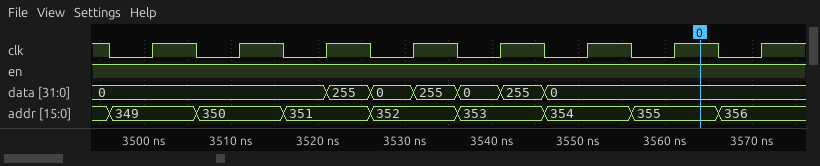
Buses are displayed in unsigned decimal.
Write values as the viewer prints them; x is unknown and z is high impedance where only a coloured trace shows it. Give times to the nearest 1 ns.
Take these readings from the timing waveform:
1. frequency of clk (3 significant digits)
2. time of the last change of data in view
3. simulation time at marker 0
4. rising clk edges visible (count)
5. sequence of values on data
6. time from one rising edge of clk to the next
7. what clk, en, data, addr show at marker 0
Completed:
100 MHz
3546 ns
3564 ns
8
0, 255, 0, 255, 0, 255, 0
10 ns
clk=1, en=1, data=0, addr=355
